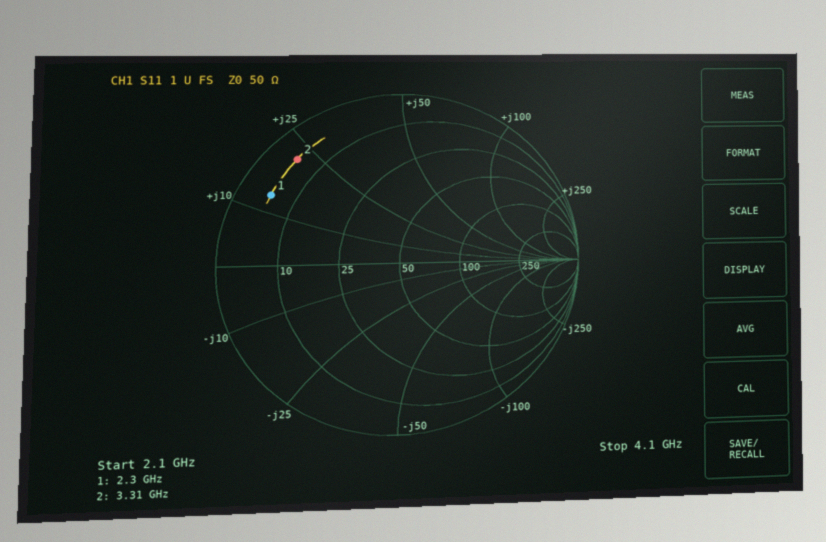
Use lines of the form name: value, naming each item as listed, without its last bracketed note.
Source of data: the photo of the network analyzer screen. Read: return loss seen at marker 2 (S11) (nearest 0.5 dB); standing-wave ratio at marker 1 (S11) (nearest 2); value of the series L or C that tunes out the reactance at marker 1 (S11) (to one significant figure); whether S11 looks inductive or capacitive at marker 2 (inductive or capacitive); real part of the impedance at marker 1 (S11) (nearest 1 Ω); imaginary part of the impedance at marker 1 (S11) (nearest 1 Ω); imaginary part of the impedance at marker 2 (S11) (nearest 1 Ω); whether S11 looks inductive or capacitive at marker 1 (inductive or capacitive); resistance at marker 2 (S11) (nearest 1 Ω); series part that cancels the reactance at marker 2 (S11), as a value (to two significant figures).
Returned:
return loss seen at marker 2 (S11): 1.5 dB
standing-wave ratio at marker 1 (S11): 10
value of the series L or C that tunes out the reactance at marker 1 (S11): 5 pF
whether S11 looks inductive or capacitive at marker 2: inductive
real part of the impedance at marker 1 (S11): 5 Ω
imaginary part of the impedance at marker 1 (S11): +13 Ω
imaginary part of the impedance at marker 2 (S11): +22 Ω
whether S11 looks inductive or capacitive at marker 1: inductive
resistance at marker 2 (S11): 5 Ω
series part that cancels the reactance at marker 2 (S11), as a value: 2.2 pF
